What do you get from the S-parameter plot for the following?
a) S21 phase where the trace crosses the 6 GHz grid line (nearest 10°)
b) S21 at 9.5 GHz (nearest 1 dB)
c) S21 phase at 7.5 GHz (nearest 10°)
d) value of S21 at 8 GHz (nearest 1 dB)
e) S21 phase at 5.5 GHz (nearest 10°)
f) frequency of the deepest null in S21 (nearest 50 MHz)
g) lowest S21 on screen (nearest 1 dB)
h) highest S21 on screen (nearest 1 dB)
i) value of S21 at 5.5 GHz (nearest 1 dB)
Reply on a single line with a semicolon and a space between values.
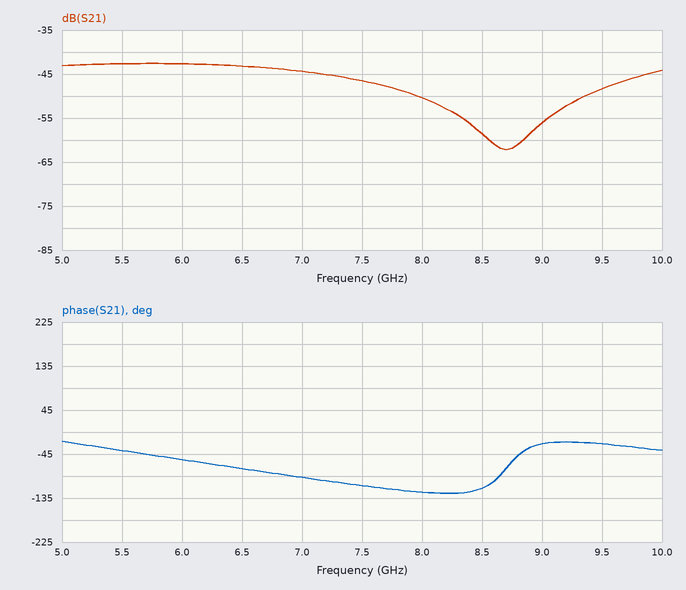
-60°; -48 dB; -110°; -50 dB; -40°; 8.70 GHz; -62 dB; -43 dB; -43 dB
